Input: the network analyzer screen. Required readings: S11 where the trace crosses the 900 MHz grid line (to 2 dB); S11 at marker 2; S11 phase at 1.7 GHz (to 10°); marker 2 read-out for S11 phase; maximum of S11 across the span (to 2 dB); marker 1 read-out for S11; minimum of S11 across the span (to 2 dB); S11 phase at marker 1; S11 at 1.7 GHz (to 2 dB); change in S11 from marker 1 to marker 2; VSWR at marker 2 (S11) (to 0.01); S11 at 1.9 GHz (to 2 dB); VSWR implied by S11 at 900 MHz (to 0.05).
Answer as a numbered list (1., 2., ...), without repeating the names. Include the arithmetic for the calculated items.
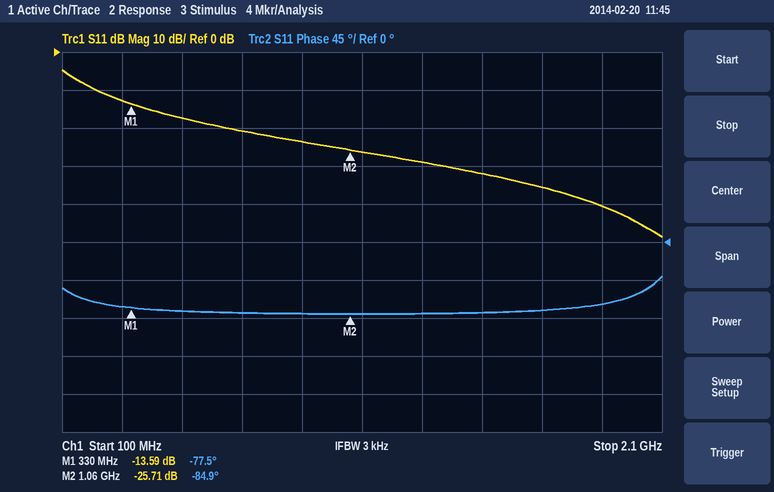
1. -24 dB
2. -25.71 dB
3. -80°
4. -84.9°
5. -4 dB
6. -13.59 dB
7. -48 dB
8. -77.5°
9. -36 dB
10. -25.71 − (-13.59) = -12.12 dB
11. (1 + 0.0518)/(1 − 0.0518) ≈ 1.11
12. -40 dB
13. |Γ| = 10^(-24/20) = 0.0631; VSWR = (1 + 0.0631)/(1 − 0.0631) ≈ 1.13, so 1.15 to the nearest 0.05
